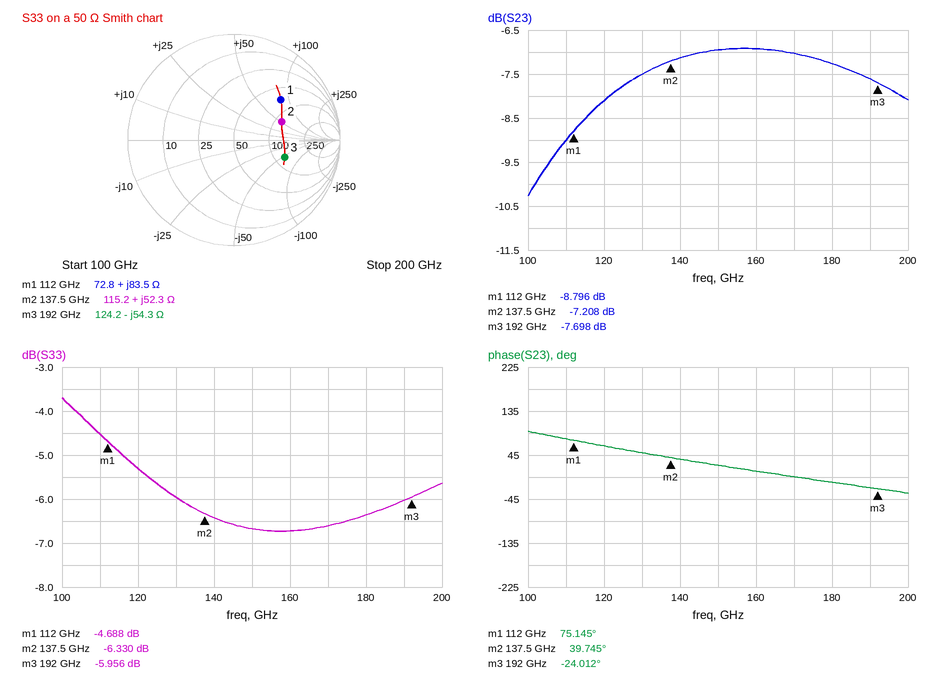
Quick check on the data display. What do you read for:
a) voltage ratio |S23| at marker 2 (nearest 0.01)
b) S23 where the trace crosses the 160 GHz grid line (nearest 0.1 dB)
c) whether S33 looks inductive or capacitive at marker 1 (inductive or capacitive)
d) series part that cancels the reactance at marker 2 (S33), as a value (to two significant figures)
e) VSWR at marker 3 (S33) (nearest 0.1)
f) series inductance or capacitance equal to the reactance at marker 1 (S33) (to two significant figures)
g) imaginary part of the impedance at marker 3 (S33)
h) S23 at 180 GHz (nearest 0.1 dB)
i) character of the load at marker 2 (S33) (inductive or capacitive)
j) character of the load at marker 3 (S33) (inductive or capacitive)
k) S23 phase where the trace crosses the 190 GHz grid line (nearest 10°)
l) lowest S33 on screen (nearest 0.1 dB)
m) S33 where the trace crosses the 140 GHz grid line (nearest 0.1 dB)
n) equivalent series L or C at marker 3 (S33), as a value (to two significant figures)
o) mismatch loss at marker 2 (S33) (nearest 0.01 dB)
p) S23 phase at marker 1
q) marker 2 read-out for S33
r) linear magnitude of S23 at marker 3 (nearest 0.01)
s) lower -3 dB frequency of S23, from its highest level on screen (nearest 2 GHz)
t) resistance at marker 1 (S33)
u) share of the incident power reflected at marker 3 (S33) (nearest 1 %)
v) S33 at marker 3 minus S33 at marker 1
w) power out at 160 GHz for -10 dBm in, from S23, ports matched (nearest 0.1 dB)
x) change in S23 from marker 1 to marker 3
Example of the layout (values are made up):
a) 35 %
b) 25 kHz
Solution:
a) 0.44
b) -6.9 dB
c) inductive
d) 22 fF
e) 3.0
f) 120 pH
g) -54.3 Ω
h) -7.3 dB
i) inductive
j) capacitive
k) -20°
l) -6.7 dB
m) -6.4 dB
n) 15 fF
o) 1.15 dB
p) 75.145°
q) -6.330 dB
r) 0.41
s) 102 GHz
t) 72.8 Ω
u) 25 %
v) -1.268 dB
w) -16.9 dBm
x) 1.098 dB
